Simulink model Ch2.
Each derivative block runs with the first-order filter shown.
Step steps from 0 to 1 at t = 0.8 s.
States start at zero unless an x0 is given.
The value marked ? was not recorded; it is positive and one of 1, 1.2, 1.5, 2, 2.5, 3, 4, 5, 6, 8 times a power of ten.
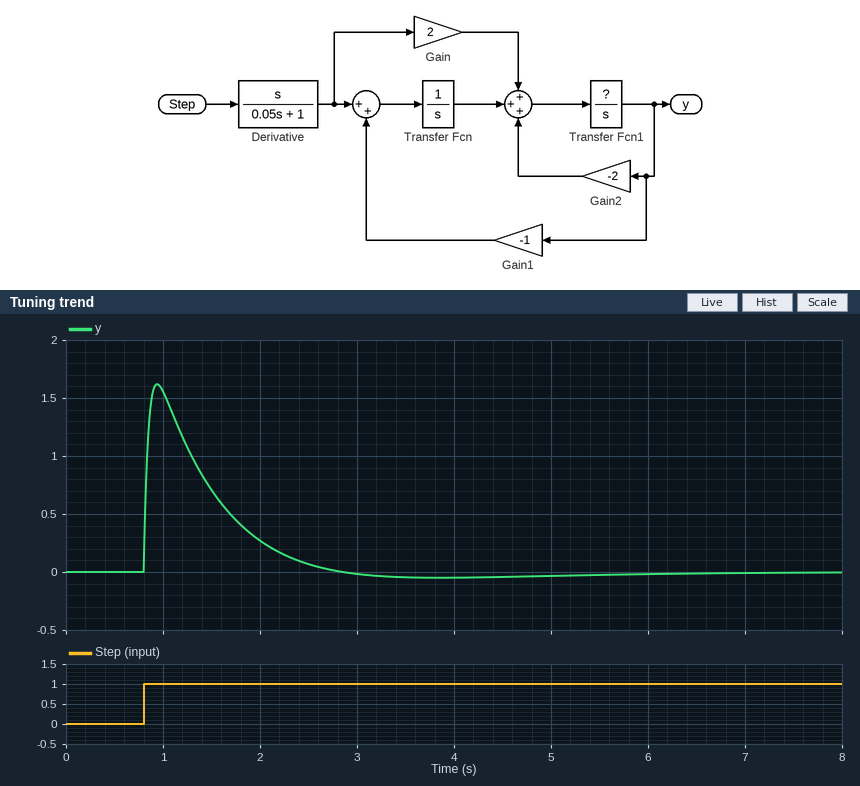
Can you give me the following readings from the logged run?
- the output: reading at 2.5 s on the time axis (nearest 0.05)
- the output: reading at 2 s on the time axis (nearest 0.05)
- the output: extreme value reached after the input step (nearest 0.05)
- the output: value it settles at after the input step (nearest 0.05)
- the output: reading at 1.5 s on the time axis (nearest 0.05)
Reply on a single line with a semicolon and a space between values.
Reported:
0.05; 0.25; 1.60; 0.00; 0.70
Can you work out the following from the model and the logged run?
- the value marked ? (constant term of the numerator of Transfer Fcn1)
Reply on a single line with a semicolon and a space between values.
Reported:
1
